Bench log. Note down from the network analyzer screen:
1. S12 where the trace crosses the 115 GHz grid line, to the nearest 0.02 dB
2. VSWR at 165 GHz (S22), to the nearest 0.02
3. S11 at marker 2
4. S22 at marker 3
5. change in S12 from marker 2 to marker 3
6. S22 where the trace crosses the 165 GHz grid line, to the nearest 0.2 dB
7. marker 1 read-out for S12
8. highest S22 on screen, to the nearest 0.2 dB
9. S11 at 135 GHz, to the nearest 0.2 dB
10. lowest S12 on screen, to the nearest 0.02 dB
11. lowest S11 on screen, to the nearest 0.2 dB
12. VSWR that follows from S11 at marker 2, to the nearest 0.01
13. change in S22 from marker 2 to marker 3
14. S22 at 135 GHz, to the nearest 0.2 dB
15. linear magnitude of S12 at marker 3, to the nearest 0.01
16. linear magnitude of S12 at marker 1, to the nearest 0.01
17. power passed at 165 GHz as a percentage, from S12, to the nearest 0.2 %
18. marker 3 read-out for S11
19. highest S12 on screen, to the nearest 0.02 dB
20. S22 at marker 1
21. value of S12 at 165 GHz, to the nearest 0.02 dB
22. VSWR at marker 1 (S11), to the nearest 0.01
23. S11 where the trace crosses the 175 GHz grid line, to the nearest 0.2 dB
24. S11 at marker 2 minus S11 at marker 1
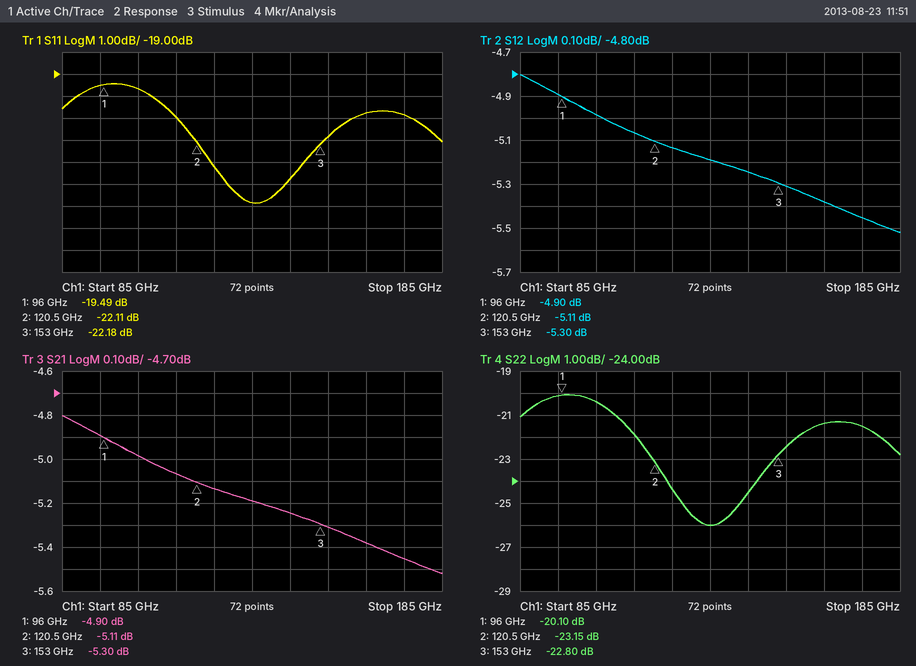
-5.06 dB
1.18
-22.11 dB
-22.80 dB
-0.19 dB
-21.4 dB
-4.90 dB
-20.0 dB
-24.8 dB
-5.52 dB
-24.8 dB
1.17
0.35 dB
-26.0 dB
0.54
0.57
29.0 %
-22.18 dB
-4.80 dB
-20.10 dB
-5.38 dB
1.24
-20.8 dB
-2.62 dB
